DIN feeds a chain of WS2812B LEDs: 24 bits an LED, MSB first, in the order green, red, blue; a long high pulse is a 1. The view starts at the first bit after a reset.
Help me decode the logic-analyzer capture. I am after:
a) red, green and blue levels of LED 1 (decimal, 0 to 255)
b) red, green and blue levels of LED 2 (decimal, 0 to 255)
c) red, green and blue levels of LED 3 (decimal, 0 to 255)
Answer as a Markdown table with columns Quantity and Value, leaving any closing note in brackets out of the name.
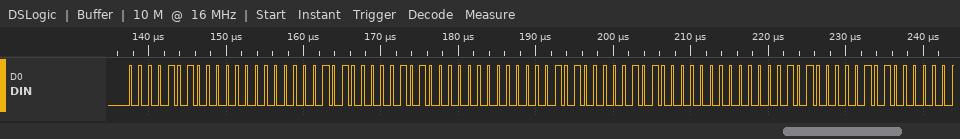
| Quantity | Value |
|---|---|
| red, green and blue levels of LED 1 | 0, 10, 10 |
| red, green and blue levels of LED 2 | 0, 10, 10 |
| red, green and blue levels of LED 3 | 0, 10, 10 |
